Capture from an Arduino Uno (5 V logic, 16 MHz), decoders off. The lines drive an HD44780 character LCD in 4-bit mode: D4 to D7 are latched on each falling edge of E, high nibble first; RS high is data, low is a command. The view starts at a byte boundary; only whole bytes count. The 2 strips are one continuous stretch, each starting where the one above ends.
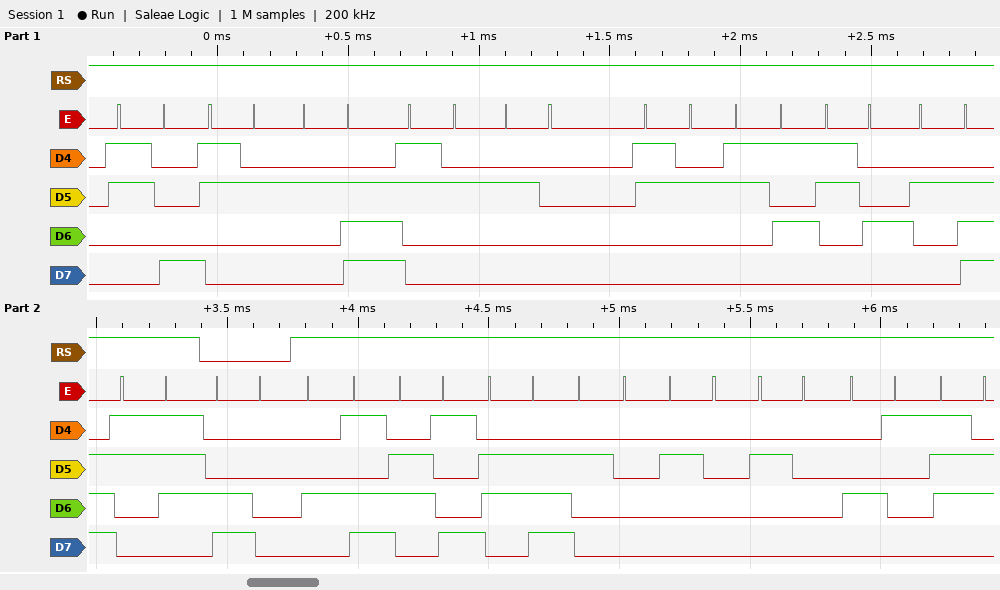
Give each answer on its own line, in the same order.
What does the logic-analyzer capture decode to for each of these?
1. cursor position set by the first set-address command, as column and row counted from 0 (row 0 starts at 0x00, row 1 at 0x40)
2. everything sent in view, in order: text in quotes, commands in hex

column 0, row 1
"82.2 254.7" 0xC0 "Min   Av"
